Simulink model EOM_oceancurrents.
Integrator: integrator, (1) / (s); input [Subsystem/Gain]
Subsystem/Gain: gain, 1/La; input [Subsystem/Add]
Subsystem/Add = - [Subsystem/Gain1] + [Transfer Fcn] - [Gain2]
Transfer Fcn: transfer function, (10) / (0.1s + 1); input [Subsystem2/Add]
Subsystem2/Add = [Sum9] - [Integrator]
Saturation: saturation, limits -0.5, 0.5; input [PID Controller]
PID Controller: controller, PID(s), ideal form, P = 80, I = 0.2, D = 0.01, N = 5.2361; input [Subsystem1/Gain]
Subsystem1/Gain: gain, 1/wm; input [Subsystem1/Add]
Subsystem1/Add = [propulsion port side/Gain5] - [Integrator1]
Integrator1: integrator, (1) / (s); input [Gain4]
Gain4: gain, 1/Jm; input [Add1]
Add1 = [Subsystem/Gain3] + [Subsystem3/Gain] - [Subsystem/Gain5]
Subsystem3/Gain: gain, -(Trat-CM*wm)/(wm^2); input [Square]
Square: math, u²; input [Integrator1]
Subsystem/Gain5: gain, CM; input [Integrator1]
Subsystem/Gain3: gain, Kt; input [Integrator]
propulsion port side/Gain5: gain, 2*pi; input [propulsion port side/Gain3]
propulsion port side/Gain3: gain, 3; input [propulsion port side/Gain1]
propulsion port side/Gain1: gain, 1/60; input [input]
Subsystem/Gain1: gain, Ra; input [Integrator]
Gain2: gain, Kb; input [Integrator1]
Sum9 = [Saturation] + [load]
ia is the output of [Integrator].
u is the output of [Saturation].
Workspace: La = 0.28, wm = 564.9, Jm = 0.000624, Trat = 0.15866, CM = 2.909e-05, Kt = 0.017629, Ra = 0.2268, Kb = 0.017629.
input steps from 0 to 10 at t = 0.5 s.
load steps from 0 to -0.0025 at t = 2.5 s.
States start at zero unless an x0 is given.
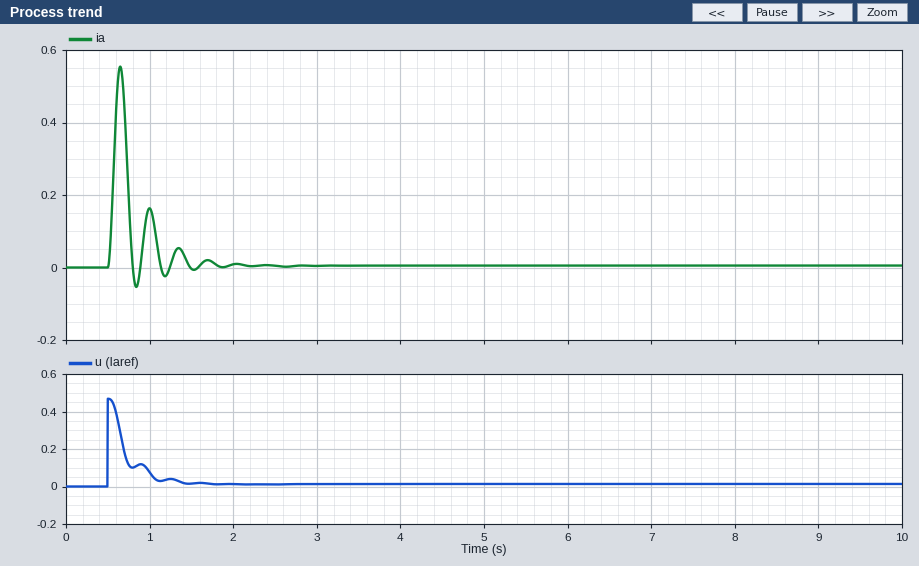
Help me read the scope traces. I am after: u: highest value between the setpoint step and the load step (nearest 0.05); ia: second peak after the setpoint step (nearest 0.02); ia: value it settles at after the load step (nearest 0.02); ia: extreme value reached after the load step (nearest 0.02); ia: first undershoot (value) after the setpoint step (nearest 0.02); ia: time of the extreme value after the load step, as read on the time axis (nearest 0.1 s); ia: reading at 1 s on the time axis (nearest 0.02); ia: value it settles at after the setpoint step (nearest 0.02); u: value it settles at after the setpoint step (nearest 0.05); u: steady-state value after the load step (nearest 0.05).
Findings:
0.45
0.16
0.00
0.00
-0.06
2.6 s
0.16
0.00
0.00
0.00
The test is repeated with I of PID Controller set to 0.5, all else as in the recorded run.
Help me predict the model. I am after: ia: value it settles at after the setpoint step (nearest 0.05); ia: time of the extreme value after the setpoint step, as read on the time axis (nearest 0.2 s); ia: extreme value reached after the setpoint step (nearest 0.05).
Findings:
0.00
0.6 s
0.55
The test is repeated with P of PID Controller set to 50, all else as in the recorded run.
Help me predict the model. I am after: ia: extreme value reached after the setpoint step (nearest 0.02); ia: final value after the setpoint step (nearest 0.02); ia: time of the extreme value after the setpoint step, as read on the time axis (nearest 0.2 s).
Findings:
0.36
0.00
0.6 s
